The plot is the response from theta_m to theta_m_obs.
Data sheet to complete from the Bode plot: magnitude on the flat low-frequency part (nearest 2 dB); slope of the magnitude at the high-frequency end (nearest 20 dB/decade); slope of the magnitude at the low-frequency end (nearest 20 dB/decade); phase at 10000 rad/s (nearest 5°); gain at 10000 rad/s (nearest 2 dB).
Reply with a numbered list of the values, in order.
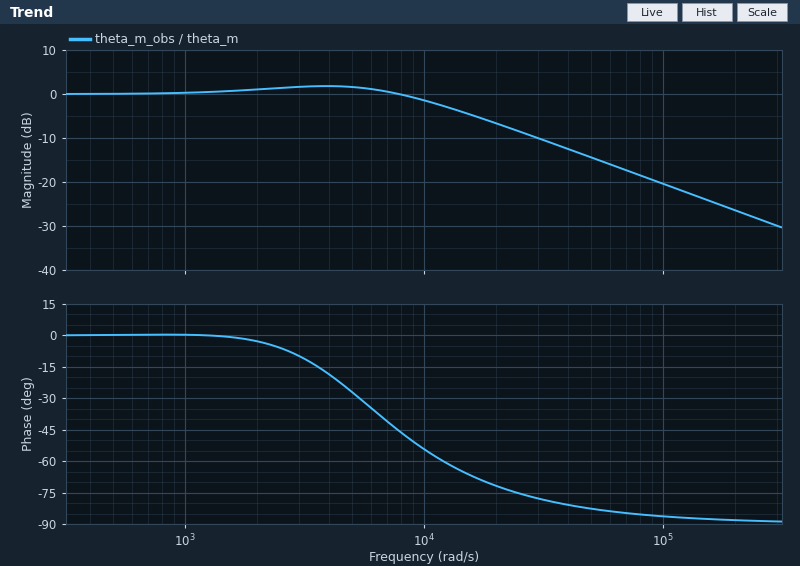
1. 0 dB
2. -20 dB/decade
3. 0 dB/decade
4. -55°
5. -2 dB
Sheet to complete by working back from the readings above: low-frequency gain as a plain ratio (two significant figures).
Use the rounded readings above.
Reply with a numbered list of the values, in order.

1. 1.0
